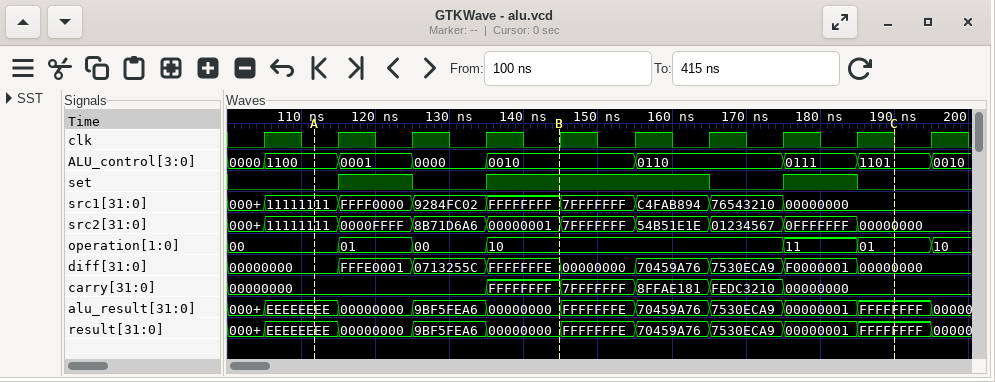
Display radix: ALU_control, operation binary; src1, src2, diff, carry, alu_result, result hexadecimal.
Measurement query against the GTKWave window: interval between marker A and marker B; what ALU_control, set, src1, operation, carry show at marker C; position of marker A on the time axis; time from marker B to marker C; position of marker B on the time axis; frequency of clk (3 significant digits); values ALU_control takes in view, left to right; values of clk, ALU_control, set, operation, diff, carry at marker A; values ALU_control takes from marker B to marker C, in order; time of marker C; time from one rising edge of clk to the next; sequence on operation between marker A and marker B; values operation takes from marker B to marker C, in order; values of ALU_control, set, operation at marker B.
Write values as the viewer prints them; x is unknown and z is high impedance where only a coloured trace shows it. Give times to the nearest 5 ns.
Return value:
35 ns
ALU_control=1101, set=0, src1=00000000, operation=01, carry=00000000
110 ns
45 ns
145 ns
100 MHz
0000, 1100, 0001, 0000, 0010, 0110, 0111, 1101, 0010
clk=0, ALU_control=1100, set=0, operation=00, diff=00000000, carry=00000000
0010, 0110, 0111, 1101
190 ns
10 ns
00, 01, 00, 10
10, 11, 01
ALU_control=0010, set=1, operation=10
